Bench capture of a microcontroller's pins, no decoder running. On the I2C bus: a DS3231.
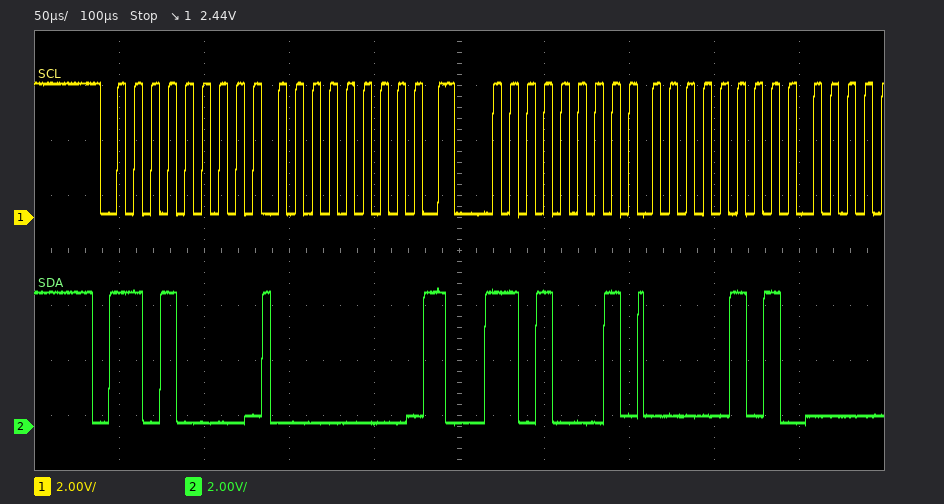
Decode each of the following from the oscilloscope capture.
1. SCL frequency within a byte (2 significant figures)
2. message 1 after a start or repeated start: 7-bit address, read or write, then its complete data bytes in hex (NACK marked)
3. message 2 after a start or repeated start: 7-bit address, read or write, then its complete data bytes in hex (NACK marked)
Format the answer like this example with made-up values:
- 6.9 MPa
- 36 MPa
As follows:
- 100 kHz
- 0x68 write: 00
- 0x68 read: 05
